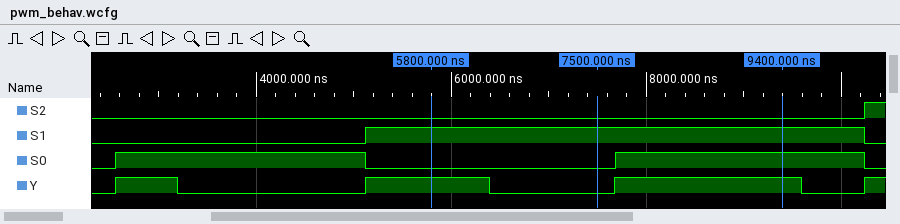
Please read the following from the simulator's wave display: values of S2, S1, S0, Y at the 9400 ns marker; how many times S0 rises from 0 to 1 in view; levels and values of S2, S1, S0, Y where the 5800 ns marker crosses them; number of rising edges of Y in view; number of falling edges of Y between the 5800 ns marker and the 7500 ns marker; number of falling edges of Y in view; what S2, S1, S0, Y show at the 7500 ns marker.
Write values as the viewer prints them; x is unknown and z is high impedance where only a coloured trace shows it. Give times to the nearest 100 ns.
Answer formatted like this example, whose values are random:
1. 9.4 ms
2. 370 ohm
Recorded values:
1. S2=0, S1=1, S0=1, Y=1
2. 2
3. S2=0, S1=1, S0=0, Y=1
4. 4
5. 1
6. 3
7. S2=0, S1=1, S0=0, Y=0
